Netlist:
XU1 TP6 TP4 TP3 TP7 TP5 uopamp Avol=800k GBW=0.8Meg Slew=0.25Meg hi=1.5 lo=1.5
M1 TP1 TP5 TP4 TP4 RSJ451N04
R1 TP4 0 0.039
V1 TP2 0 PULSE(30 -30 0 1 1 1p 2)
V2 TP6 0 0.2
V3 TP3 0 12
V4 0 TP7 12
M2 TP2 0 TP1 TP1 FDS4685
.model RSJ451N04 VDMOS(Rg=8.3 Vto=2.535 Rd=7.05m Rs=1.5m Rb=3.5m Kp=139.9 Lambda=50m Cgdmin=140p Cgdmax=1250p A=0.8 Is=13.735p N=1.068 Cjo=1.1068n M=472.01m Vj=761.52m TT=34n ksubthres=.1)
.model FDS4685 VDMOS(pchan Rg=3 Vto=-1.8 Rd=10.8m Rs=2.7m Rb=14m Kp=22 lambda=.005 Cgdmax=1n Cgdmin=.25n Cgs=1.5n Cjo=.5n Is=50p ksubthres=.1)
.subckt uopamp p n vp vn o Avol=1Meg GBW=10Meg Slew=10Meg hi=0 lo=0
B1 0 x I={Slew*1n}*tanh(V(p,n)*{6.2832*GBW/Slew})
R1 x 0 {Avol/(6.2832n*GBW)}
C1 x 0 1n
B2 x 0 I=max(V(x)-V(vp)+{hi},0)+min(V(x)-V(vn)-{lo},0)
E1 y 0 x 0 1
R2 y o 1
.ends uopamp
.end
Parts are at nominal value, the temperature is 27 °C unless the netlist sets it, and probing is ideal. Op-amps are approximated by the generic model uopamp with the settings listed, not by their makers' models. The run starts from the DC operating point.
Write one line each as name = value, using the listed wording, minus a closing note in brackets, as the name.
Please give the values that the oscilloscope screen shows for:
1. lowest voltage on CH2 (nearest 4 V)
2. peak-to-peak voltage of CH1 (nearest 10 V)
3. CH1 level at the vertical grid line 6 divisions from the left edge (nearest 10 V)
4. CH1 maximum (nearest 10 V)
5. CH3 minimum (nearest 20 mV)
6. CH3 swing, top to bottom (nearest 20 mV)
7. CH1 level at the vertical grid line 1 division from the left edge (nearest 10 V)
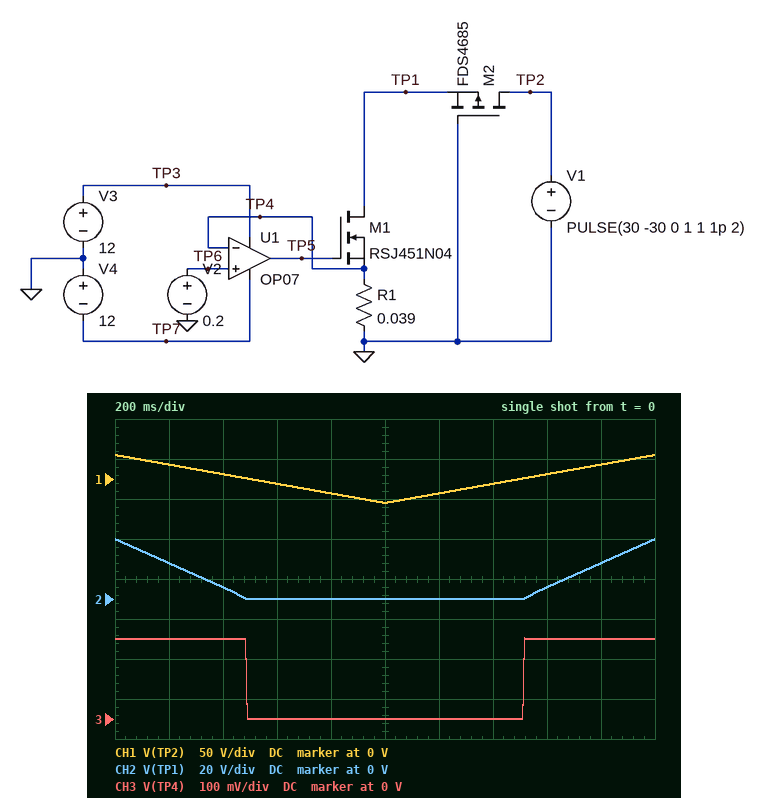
lowest voltage on CH2 = 0 V
peak-to-peak voltage of CH1 = 60 V
CH1 level at the vertical grid line 6 divisions from the left edge = -20 V
CH1 maximum = 30 V
CH3 minimum = 0 V
CH3 swing, top to bottom = 200 mV
CH1 level at the vertical grid line 1 division from the left edge = 20 V
